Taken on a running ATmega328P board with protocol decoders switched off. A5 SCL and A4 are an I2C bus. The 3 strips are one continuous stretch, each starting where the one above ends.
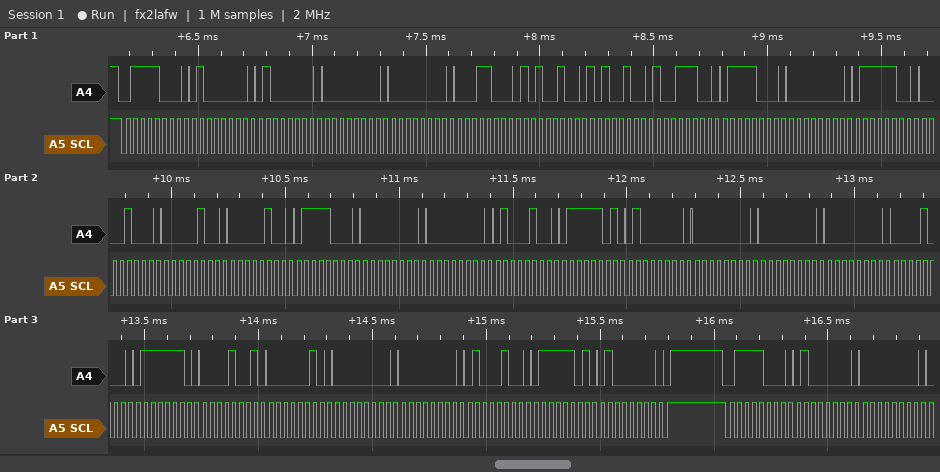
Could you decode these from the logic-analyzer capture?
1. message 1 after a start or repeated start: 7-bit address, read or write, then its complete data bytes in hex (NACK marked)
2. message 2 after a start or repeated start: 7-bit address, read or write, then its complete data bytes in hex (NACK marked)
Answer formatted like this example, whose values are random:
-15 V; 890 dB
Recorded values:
0x3C write: 40 40 00 00 18 A4 A4 9C 78 00 7C 08 04 04 78 00 00 44 7D 40 00 00 00 08 7E 09 02 00 00 44 7D 40; 0x3C write: 40 00
